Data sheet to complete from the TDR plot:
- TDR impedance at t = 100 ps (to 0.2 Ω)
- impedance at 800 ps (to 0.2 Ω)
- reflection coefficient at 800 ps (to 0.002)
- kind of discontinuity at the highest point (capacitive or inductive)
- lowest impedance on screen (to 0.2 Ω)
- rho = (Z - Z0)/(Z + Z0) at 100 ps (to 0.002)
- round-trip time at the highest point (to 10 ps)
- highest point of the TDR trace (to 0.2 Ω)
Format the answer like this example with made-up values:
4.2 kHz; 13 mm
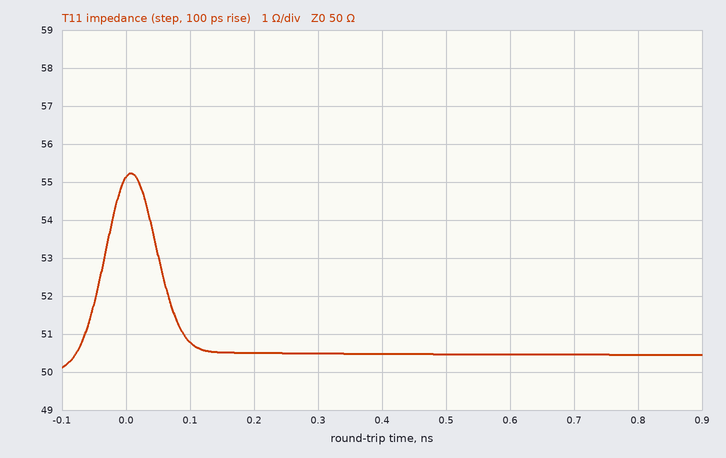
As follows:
50.8 Ω; 50.4 Ω; +0.004; inductive; 50.2 Ω; +0.008; 10 ps; 55.2 Ω
